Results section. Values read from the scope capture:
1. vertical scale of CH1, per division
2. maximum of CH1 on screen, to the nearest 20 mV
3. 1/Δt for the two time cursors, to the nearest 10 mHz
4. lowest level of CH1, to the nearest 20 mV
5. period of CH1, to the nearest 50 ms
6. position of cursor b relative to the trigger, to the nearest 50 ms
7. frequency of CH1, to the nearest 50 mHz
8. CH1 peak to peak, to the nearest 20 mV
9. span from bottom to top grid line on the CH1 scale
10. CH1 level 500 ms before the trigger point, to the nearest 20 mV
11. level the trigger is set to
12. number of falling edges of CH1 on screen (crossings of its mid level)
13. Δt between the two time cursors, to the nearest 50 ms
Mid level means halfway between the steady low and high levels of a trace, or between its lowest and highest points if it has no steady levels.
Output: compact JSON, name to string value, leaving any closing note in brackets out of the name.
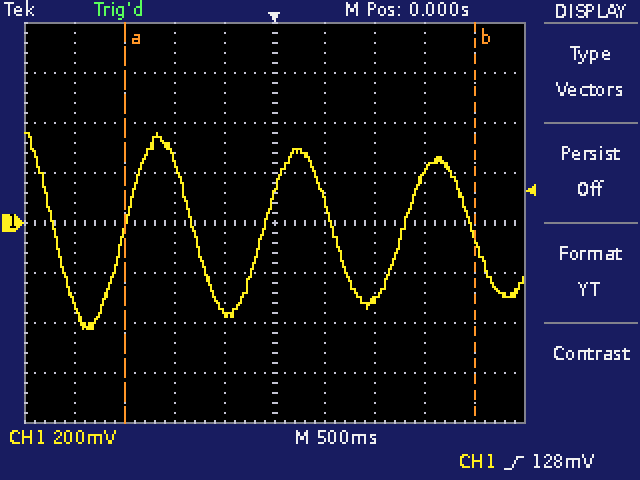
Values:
{"vertical scale of CH1, per division": "200 mV", "maximum of CH1 on screen, to the nearest 20 mV": "360 mV", "1/Δt for the two time cursors, to the nearest 10 mHz": "290 mHz", "lowest level of CH1, to the nearest 20 mV": "-420 mV", "period of CH1, to the nearest 50 ms": "1.40 s", "position of cursor b relative to the trigger, to the nearest 50 ms": "+2.00 s", "frequency of CH1, to the nearest 50 mHz": "700 mHz", "CH1 peak to peak, to the nearest 20 mV": "780 mV", "span from bottom to top grid line on the CH1 scale": "1.6 V", "CH1 level 500 ms before the trigger point, to the nearest 20 mV": "-360 mV", "level the trigger is set to": "128 mV", "number of falling edges of CH1 on screen": "4", "Δt between the two time cursors, to the nearest 50 ms": "3.50 s"}
